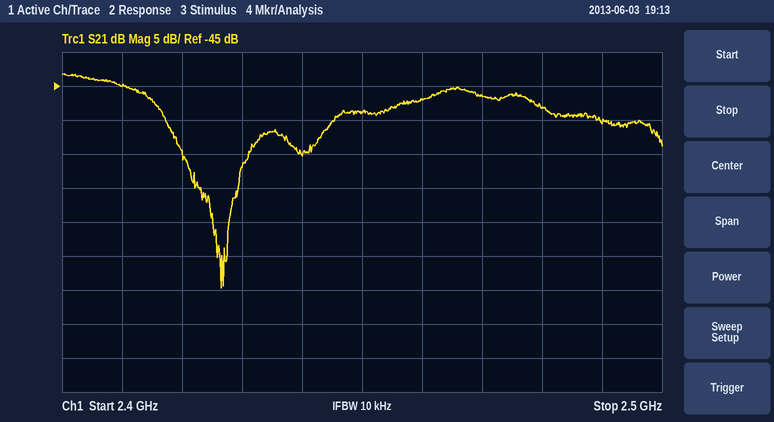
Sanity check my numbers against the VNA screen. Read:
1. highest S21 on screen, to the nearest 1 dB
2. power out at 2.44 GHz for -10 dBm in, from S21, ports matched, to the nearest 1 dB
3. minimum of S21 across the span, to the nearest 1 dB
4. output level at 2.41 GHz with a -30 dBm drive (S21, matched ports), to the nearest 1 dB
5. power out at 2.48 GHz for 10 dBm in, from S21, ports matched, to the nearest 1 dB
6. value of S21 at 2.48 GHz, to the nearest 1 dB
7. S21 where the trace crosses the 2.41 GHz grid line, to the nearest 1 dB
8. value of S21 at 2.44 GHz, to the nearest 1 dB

-43 dB
-65 dBm
-75 dB
-75 dBm
-38 dBm
-48 dB
-45 dB
-55 dB
